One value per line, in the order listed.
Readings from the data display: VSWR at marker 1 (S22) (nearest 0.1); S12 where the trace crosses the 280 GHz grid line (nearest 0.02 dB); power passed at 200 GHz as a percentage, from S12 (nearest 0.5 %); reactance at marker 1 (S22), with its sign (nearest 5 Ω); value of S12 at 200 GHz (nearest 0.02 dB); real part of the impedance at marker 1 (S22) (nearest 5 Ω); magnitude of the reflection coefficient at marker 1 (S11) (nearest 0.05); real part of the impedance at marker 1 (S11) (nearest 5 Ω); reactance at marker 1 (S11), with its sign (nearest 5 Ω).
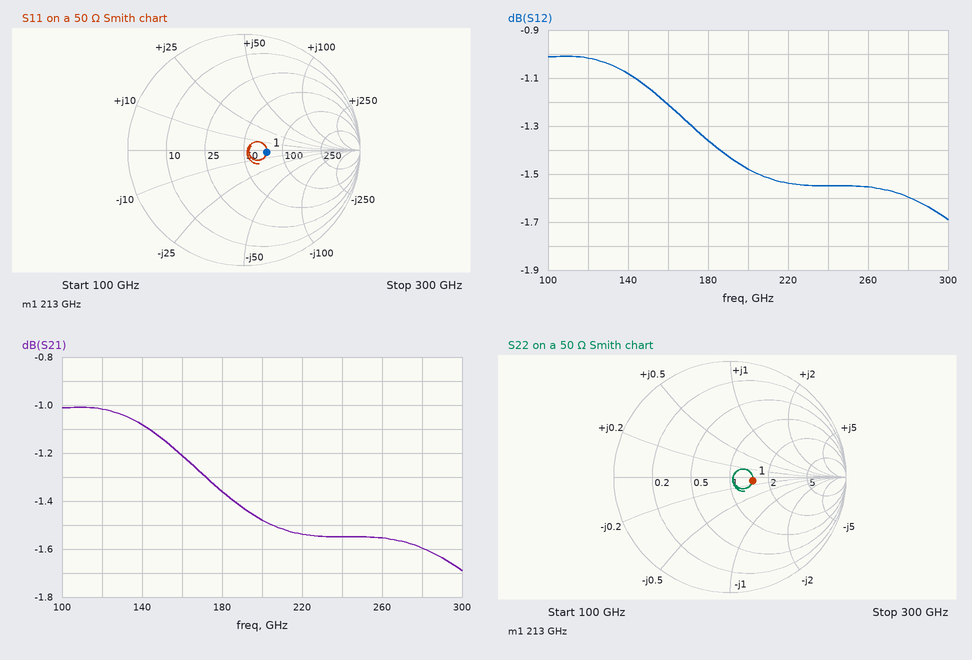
1.5
-1.60 dB
71.0 %
-5 Ω
-1.48 dB
75 Ω
0.20
75 Ω
-5 Ω
